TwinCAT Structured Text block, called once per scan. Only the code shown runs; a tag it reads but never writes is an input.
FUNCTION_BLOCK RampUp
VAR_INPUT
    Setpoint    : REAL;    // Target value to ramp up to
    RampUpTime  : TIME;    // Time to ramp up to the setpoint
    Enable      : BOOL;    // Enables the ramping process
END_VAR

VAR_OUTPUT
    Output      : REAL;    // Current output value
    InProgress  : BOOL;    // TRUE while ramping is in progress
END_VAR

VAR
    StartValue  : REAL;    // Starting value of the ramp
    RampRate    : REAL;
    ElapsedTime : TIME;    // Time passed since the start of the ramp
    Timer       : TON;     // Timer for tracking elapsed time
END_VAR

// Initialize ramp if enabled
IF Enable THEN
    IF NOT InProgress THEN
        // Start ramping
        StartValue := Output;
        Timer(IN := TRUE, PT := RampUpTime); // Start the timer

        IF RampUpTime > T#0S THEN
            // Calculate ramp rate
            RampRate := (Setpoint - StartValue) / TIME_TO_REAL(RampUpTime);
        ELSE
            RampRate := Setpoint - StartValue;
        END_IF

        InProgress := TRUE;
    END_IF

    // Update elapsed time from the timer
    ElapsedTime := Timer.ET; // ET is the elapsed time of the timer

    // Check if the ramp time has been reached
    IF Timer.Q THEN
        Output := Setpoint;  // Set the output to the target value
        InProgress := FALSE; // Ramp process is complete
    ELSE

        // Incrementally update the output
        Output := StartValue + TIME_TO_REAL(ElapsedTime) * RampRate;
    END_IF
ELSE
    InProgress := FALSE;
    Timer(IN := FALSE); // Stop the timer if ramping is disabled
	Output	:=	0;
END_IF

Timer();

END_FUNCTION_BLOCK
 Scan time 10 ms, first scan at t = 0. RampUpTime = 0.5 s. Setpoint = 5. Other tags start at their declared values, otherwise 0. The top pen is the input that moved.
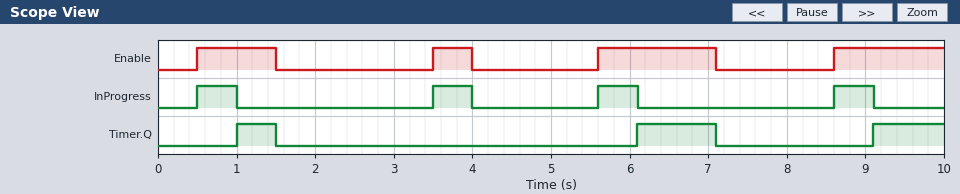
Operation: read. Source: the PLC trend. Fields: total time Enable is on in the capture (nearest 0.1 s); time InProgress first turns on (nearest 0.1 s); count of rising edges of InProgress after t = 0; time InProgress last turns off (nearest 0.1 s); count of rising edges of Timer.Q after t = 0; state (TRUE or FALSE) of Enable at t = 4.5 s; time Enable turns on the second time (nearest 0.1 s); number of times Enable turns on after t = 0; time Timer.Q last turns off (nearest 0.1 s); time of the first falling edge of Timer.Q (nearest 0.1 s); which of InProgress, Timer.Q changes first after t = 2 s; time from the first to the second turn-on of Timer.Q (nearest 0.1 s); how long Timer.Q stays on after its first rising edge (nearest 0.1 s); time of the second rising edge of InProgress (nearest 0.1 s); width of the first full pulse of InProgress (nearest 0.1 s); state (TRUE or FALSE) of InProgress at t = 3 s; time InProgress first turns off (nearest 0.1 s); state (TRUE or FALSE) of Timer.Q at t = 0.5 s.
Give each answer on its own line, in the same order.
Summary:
4.4 s
0.5 s
4
9.1 s
3
FALSE
3.5 s
4
7.1 s
1.5 s
InProgress
5.1 s
0.5 s
3.5 s
0.5 s
FALSE
1.0 s
FALSE
